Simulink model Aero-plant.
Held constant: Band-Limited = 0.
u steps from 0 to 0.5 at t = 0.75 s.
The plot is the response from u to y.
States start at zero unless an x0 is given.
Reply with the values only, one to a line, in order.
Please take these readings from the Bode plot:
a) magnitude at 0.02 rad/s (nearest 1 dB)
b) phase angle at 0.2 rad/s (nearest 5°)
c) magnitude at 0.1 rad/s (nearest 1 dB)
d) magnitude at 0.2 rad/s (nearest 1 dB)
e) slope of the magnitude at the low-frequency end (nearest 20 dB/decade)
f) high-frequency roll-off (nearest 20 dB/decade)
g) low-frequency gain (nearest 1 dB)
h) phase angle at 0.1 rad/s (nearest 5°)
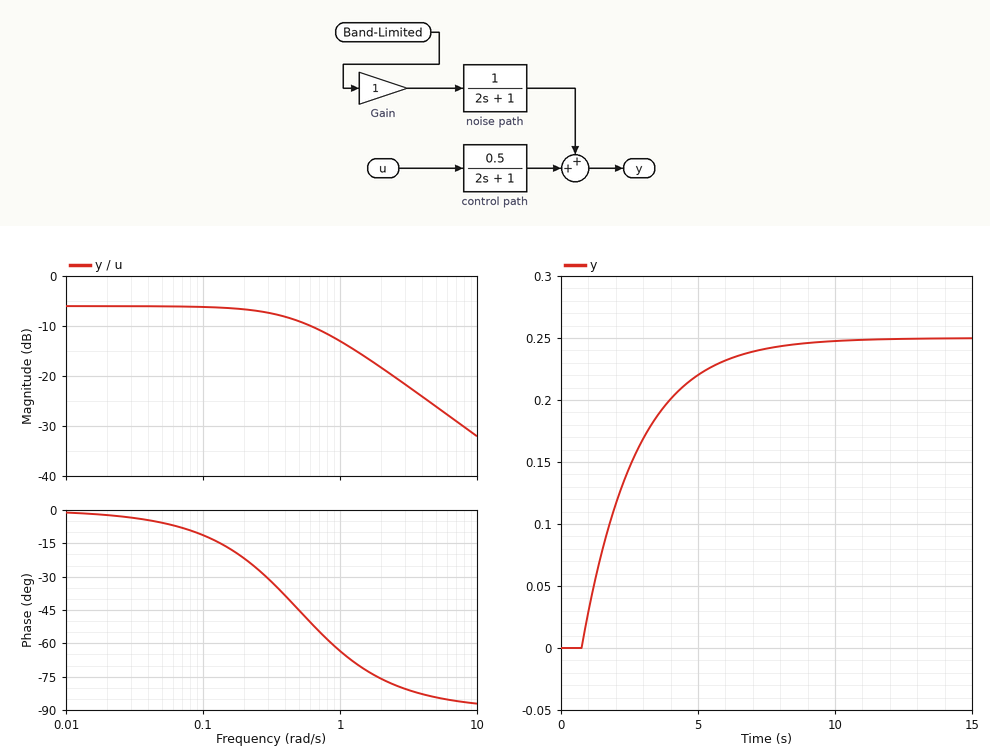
-6 dB
-20°
-6 dB
-7 dB
0 dB/decade
-20 dB/decade
-6 dB
-10°
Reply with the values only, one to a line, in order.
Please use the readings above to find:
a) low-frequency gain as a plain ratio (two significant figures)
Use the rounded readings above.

0.50
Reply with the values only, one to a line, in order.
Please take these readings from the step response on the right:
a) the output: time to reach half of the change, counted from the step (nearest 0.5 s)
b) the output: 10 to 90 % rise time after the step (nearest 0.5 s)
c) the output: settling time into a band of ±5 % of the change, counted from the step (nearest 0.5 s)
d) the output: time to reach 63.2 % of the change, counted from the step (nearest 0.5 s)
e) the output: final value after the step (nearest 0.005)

1.5 s
4.5 s
6.0 s
2.0 s
0.250
